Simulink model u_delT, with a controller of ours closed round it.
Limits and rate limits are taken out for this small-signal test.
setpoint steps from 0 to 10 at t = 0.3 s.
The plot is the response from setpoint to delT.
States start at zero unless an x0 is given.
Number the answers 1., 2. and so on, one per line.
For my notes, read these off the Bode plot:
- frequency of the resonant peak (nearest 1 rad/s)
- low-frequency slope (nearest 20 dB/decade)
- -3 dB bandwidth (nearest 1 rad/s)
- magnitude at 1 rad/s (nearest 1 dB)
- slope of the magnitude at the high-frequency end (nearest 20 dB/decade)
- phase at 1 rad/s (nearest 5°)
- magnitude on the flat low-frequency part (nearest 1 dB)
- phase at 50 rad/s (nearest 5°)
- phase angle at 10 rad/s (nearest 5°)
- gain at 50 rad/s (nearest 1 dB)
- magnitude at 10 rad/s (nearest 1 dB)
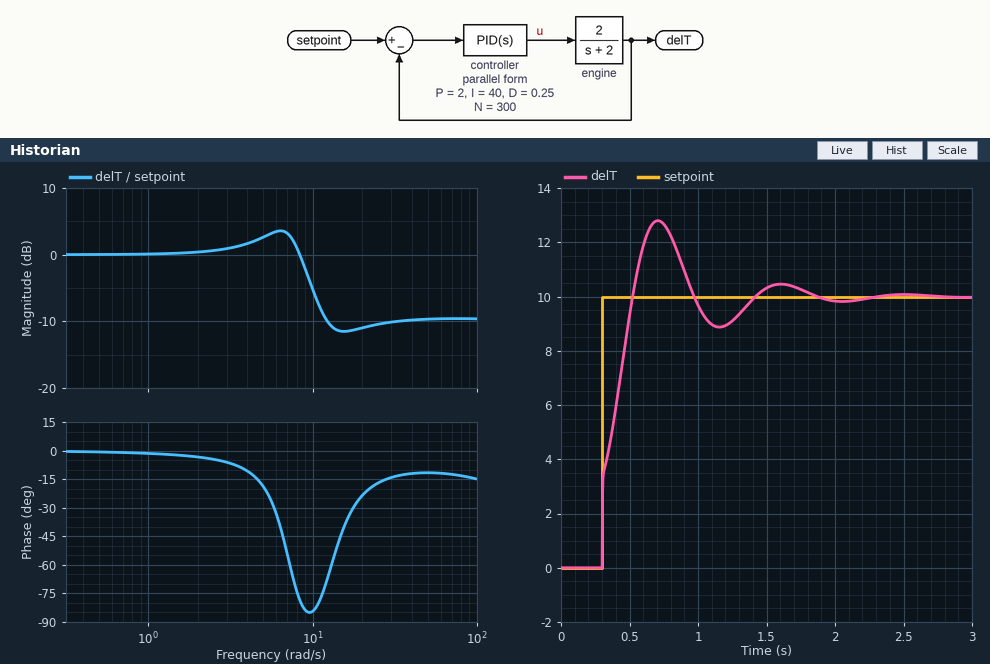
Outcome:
1. 6 rad/s
2. 0 dB/decade
3. 9 rad/s
4. 0 dB
5. 0 dB/decade
6. 0°
7. 0 dB
8. -10°
9. -85°
10. -10 dB
11. -5 dB
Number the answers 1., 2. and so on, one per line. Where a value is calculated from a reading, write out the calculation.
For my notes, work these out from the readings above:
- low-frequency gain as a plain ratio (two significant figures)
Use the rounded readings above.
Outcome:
1. 10^(0 / 20) = 1.0
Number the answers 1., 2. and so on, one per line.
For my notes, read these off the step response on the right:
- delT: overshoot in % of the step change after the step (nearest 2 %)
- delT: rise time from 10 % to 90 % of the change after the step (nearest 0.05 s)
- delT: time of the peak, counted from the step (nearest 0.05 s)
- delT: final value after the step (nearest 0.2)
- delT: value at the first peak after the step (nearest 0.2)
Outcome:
1. 28 %
2. 0.20 s
3. 0.40 s
4. 10.0
5. 12.8
